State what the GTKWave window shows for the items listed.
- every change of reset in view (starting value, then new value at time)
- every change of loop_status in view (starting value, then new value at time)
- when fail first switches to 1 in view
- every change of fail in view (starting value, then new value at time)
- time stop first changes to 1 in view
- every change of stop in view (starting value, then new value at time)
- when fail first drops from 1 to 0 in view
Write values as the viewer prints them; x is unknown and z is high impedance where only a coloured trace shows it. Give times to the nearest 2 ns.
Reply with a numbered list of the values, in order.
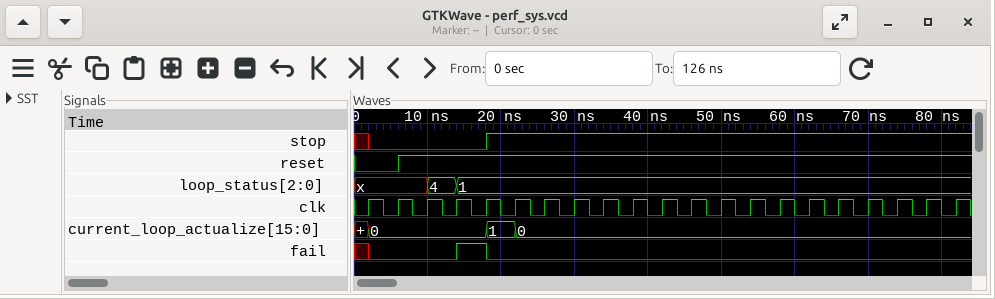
1. 0, 1 at 6 ns
2. x, 4 at 10 ns, 1 at 14 ns
3. 14 ns
4. x, 0 at 2 ns, 1 at 14 ns, 0 at 18 ns
5. 18 ns
6. x, 0 at 2 ns, 1 at 18 ns
7. 18 ns
